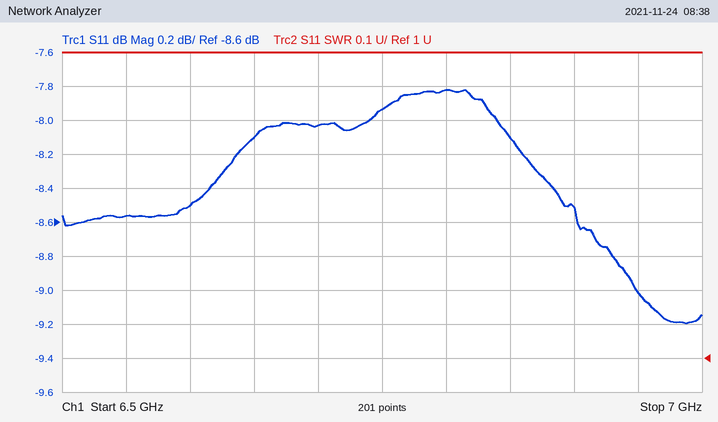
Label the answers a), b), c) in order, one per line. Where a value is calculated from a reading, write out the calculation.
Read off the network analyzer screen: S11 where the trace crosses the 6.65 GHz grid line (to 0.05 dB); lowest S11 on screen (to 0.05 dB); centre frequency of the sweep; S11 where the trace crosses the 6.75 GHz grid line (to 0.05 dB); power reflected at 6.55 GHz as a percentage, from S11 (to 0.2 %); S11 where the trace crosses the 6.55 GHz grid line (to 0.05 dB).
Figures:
a) -8.10 dB
b) -9.20 dB
c) 6.75 GHz
d) -7.95 dB
e) 10^(-8.55/10) ≈ 14.0 %
f) -8.55 dB
